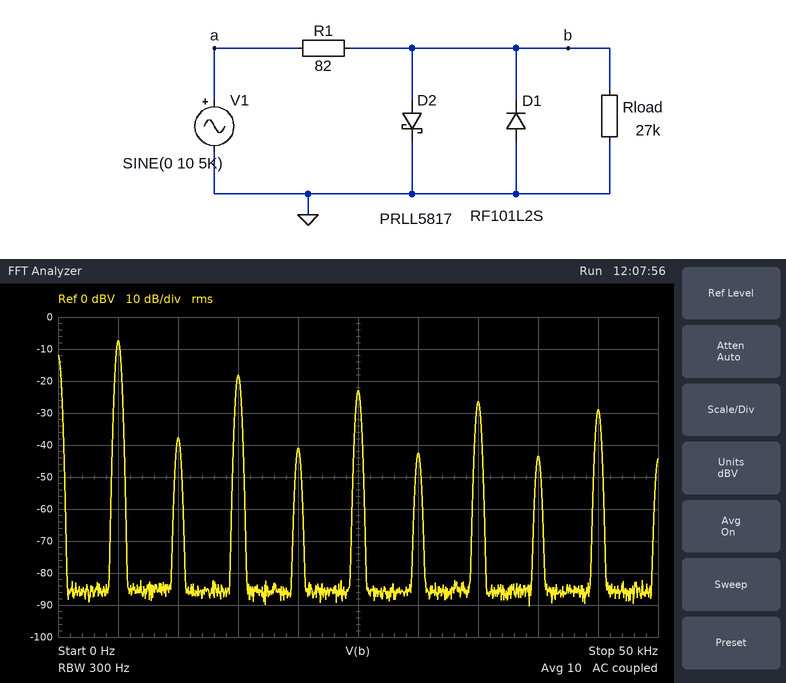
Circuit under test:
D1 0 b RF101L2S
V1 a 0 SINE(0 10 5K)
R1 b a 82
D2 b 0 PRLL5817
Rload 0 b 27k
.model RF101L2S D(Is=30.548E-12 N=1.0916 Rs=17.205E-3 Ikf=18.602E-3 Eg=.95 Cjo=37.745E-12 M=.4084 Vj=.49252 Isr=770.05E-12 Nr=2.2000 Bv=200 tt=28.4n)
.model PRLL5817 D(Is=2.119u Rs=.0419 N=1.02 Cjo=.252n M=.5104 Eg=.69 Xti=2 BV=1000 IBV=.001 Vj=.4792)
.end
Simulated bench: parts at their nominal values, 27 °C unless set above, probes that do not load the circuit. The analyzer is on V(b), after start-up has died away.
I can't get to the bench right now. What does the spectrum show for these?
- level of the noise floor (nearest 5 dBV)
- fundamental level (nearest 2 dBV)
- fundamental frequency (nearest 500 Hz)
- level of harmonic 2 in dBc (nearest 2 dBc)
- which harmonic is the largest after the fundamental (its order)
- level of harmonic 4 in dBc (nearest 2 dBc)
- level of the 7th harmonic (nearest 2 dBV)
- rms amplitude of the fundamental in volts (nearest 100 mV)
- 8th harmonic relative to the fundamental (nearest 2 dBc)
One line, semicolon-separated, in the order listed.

-85 dBV; -8 dBV; 5.0 kHz; -30 dBc; 3; -34 dBc; -26 dBV; 400 mV; -36 dBc
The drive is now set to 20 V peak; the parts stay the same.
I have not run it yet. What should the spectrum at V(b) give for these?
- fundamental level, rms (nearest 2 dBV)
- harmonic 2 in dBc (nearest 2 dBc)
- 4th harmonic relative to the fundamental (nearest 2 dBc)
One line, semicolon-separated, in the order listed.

-6 dBV; -32 dBc; -36 dBc
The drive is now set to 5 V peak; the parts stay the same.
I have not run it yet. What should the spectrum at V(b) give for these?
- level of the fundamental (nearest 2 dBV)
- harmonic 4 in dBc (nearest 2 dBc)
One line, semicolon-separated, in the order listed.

-8 dBV; -30 dBc
